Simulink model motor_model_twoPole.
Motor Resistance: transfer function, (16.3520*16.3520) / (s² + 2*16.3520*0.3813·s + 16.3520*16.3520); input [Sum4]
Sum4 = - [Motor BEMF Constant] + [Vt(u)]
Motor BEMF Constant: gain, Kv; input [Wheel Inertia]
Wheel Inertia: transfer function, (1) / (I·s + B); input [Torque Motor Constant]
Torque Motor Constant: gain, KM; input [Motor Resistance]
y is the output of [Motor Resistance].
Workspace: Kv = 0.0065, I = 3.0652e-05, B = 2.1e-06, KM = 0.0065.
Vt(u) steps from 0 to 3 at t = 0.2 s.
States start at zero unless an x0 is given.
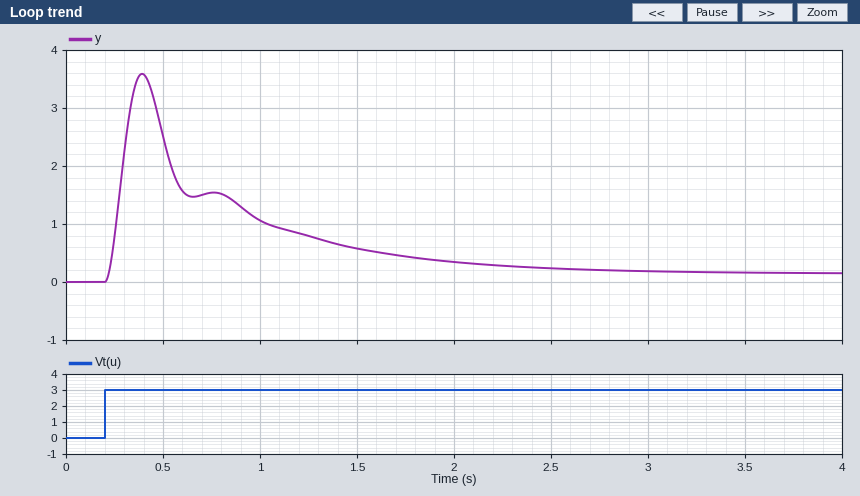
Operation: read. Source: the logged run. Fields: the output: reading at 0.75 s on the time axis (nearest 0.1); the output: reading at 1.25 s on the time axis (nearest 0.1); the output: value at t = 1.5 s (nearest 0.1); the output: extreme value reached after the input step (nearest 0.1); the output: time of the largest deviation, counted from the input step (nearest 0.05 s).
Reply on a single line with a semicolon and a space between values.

1.5; 0.8; 0.6; 3.6; 0.20 s
